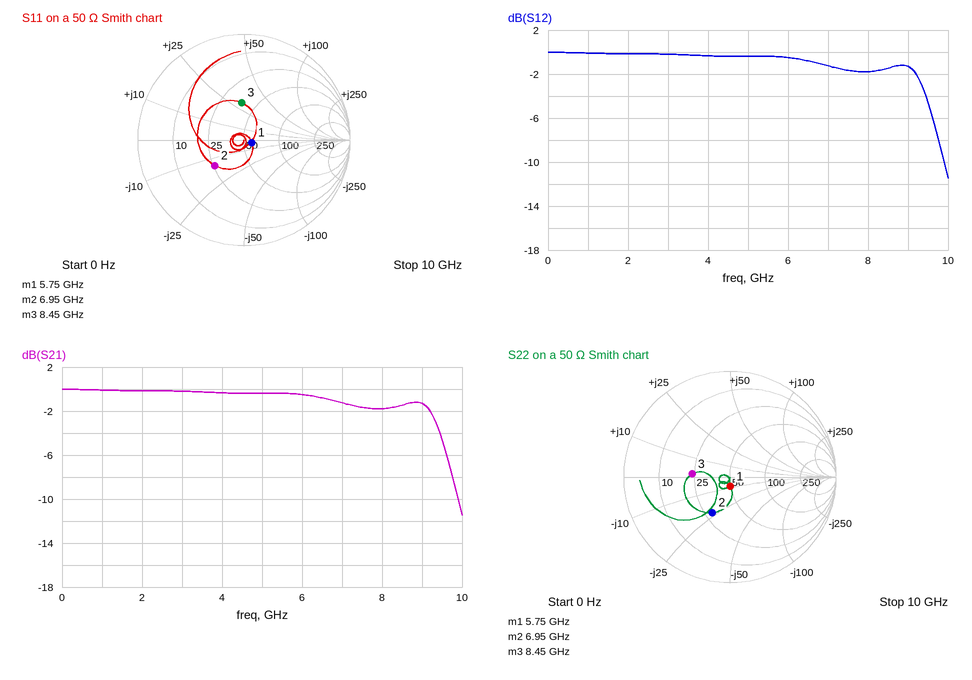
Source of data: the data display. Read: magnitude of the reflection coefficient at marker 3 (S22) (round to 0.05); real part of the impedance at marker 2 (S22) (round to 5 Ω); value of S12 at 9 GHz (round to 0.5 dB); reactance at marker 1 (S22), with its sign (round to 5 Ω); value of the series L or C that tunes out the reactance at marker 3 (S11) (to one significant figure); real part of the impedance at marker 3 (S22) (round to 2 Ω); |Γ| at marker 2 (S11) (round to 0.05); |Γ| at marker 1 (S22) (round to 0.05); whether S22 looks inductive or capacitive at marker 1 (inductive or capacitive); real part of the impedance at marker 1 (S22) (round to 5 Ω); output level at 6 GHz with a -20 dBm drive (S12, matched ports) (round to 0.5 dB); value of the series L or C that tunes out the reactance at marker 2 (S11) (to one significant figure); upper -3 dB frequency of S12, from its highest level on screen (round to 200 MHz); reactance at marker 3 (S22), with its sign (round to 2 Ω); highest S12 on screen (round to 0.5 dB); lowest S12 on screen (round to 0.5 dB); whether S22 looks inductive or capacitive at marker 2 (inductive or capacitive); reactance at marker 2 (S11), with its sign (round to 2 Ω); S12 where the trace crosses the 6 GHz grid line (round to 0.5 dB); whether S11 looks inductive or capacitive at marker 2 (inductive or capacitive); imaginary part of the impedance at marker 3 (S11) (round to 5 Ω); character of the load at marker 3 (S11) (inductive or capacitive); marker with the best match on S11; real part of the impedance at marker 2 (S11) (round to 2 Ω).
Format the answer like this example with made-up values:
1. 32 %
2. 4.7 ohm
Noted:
1. 0.35
2. 30 Ω
3. -1.5 dB
4. -10 Ω
5. 600 fF
6. 24 Ω
7. 0.35
8. 0.10
9. capacitive
10. 50 Ω
11. -20.5 dBm
12. 300 pH
13. 9.4 GHz
14. +2 Ω
15. 0.0 dB
16. -11.5 dB
17. capacitive
18. -14 Ω
19. -0.5 dB
20. capacitive
21. +30 Ω
22. inductive
23. marker 1
24. 26 Ω
